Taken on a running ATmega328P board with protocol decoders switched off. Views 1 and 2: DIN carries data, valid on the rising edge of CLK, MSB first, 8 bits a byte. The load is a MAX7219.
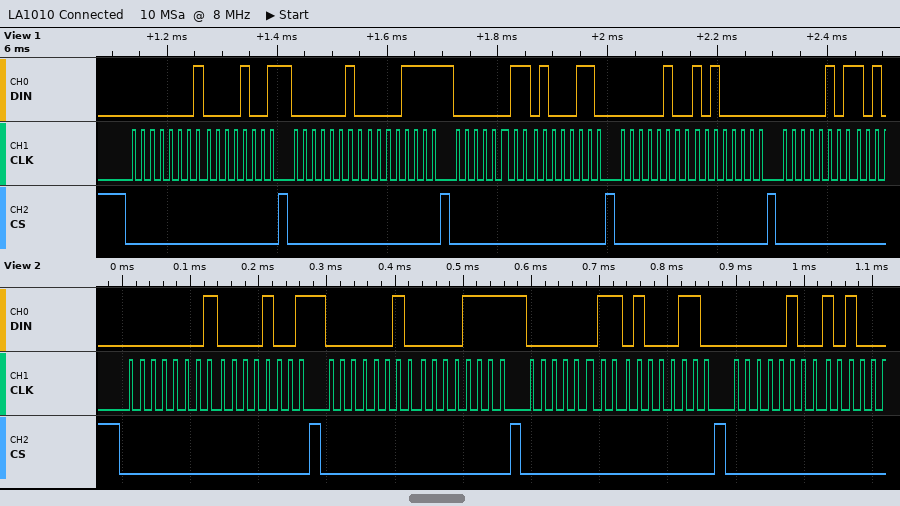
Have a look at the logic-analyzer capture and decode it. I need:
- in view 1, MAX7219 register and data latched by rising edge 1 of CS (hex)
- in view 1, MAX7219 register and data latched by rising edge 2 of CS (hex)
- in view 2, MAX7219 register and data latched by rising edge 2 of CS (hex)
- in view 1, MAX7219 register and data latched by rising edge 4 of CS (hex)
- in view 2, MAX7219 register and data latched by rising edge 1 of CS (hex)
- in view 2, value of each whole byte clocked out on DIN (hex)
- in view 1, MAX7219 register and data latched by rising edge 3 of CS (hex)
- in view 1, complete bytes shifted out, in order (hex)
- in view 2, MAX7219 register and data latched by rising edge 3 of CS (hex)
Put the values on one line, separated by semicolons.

register 0x1, data 0x09; register 0x2, data 0x0F; register 0x2, data 0x0F; register 0x4, data 0xA0; register 0x1, data 0x09; 01 09 02 0F 03 46 04; register 0x3, data 0x46; 0x01 0x09 0x02 0x0F 0x03 0x46 0x04 0xA0 0x05; register 0x3, data 0x46
